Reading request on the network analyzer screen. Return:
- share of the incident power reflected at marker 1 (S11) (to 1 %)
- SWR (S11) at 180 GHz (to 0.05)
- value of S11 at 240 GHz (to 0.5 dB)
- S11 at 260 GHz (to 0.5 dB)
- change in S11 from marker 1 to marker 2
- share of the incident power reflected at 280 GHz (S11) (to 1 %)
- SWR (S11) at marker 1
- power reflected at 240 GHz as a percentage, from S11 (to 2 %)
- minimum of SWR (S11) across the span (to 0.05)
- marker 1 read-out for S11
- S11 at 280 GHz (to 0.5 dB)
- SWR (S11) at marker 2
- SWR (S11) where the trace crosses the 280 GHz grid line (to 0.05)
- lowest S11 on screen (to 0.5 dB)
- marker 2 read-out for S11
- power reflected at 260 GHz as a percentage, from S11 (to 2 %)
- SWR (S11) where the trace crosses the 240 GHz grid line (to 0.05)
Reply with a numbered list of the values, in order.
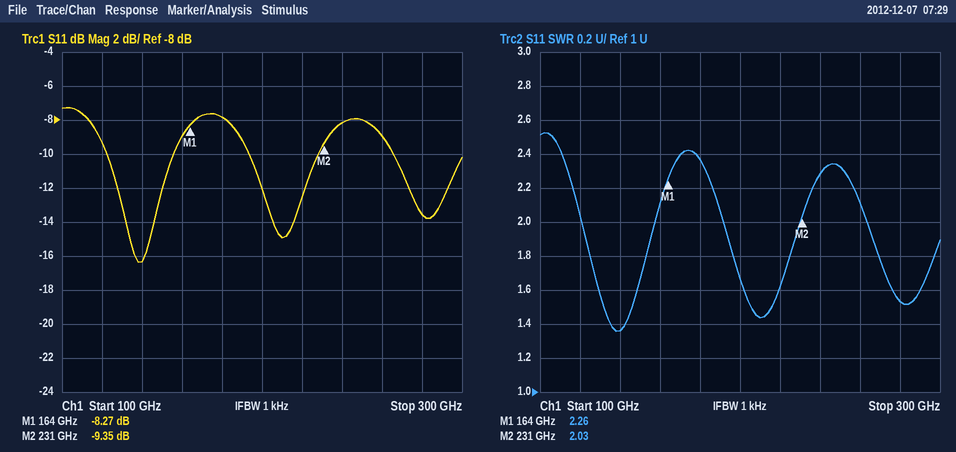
1. 15 %
2. 2.35
3. -8.0 dB
4. -9.0 dB
5. -1.08 dB
6. 4 %
7. 2.26
8. 16 %
9. 1.35
10. -8.27 dB
11. -13.5 dB
12. 2.03
13. 1.55
14. -16.5 dB
15. -9.35 dB
16. 12 %
17. 2.30
